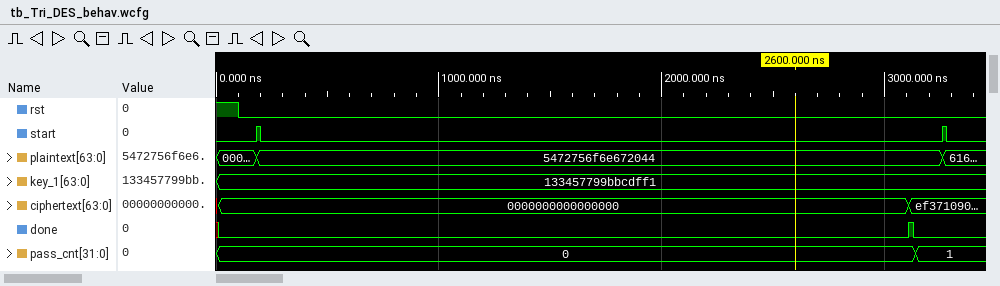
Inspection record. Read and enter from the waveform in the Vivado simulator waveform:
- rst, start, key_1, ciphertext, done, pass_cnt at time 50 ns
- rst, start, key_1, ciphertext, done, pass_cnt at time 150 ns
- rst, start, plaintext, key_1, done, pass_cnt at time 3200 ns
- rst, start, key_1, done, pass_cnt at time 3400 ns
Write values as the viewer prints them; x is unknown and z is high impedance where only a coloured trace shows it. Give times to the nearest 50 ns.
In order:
rst=1, start=0, key_1=133457799bbcdff1, ciphertext=0000000000000000, done=0, pass_cnt=0
rst=0, start=0, key_1=133457799bbcdff1, ciphertext=0000000000000000, done=0, pass_cnt=0
rst=0, start=0, plaintext=5472756f6e672044, key_1=133457799bbcdff1, done=0, pass_cnt=1
rst=0, start=0, key_1=133457799bbcdff1, done=0, pass_cnt=1
